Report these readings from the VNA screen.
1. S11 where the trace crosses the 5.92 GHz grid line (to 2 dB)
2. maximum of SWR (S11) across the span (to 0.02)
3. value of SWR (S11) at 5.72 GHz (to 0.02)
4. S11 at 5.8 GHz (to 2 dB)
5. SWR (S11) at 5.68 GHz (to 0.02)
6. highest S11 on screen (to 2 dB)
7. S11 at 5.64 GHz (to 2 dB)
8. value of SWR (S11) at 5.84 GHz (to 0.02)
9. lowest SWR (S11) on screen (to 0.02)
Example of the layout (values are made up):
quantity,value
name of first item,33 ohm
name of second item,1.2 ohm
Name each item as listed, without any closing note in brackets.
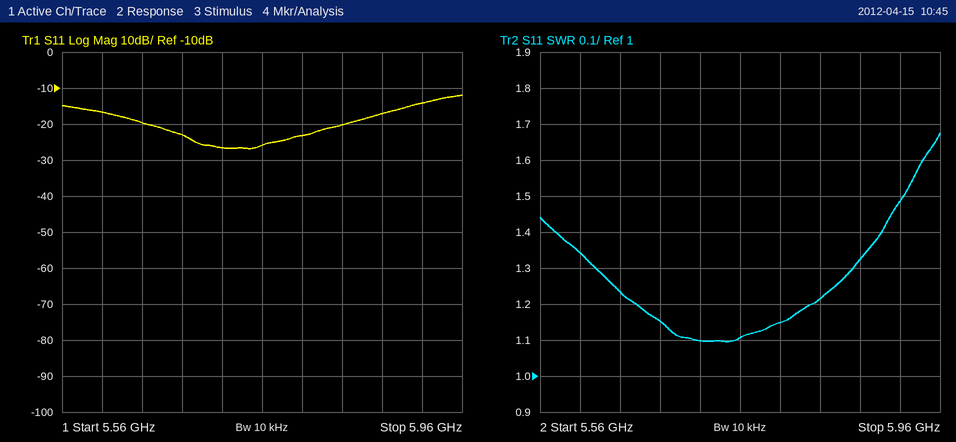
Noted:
quantity,value
S11 where the trace crosses the 5.92 GHz grid line,-14 dB
maximum of SWR (S11) across the span,1.68
value of SWR (S11) at 5.72 GHz,1.10
S11 at 5.8 GHz,-24 dB
SWR (S11) at 5.68 GHz,1.16
highest S11 on screen,-12 dB
S11 at 5.64 GHz,-20 dB
value of SWR (S11) at 5.84 GHz,1.22
lowest SWR (S11) on screen,1.10
